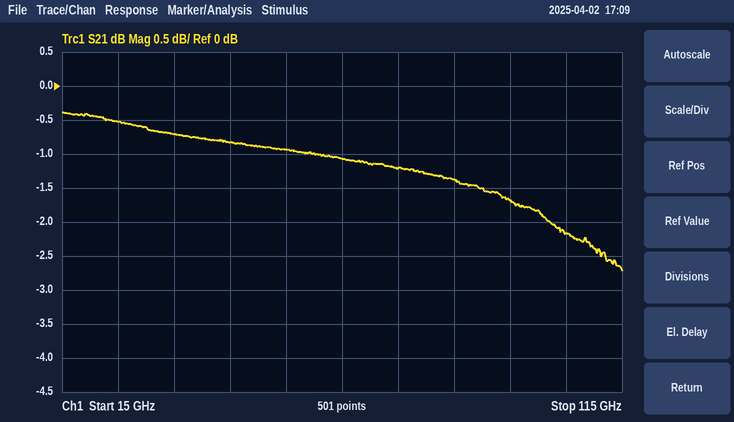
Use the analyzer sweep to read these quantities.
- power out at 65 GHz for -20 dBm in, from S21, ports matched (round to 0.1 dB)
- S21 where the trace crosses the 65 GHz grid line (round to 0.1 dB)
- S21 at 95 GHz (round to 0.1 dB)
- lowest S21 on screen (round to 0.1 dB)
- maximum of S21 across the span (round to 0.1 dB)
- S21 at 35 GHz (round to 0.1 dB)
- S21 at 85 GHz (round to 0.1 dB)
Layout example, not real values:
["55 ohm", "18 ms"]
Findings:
["-21.1 dBm", "-1.1 dB", "-1.7 dB", "-2.7 dB", "-0.4 dB", "-0.7 dB", "-1.4 dB"]
